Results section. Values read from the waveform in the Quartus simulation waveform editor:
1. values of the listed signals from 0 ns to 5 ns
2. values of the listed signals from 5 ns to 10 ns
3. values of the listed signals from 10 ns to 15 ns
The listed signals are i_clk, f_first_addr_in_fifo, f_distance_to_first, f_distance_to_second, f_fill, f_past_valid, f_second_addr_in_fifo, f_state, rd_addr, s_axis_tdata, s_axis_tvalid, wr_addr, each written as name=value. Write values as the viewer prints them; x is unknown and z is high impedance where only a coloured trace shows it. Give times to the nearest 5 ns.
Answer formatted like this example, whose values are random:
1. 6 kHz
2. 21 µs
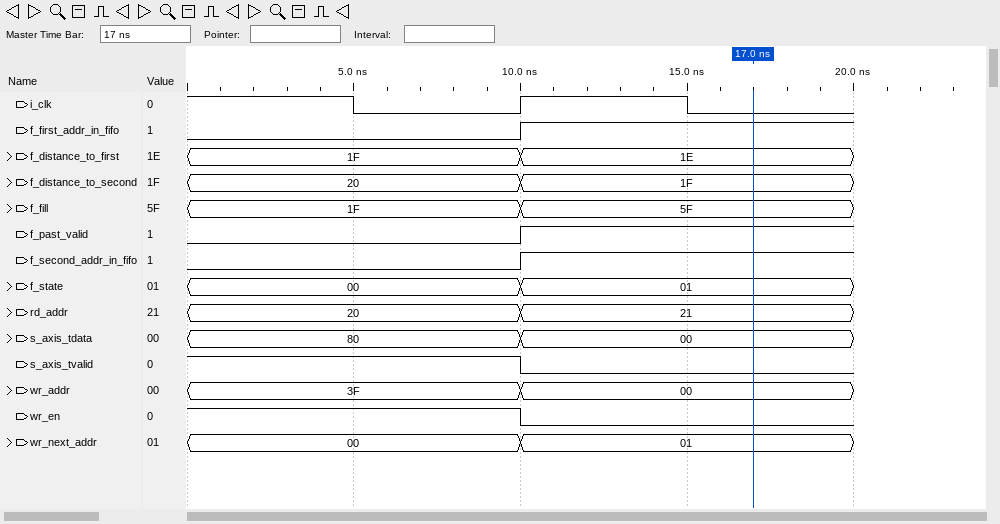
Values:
1. i_clk=1, f_first_addr_in_fifo=0, f_distance_to_first=1F, f_distance_to_second=20, f_fill=1F, f_past_valid=0, f_second_addr_in_fifo=0, f_state=00, rd_addr=20, s_axis_tdata=80, s_axis_tvalid=1, wr_addr=3F
2. i_clk=0, f_first_addr_in_fifo=0, f_distance_to_first=1F, f_distance_to_second=20, f_fill=1F, f_past_valid=0, f_second_addr_in_fifo=0, f_state=00, rd_addr=20, s_axis_tdata=80, s_axis_tvalid=1, wr_addr=3F
3. i_clk=1, f_first_addr_in_fifo=1, f_distance_to_first=1E, f_distance_to_second=1F, f_fill=5F, f_past_valid=1, f_second_addr_in_fifo=1, f_state=01, rd_addr=21, s_axis_tdata=00, s_axis_tvalid=0, wr_addr=00
